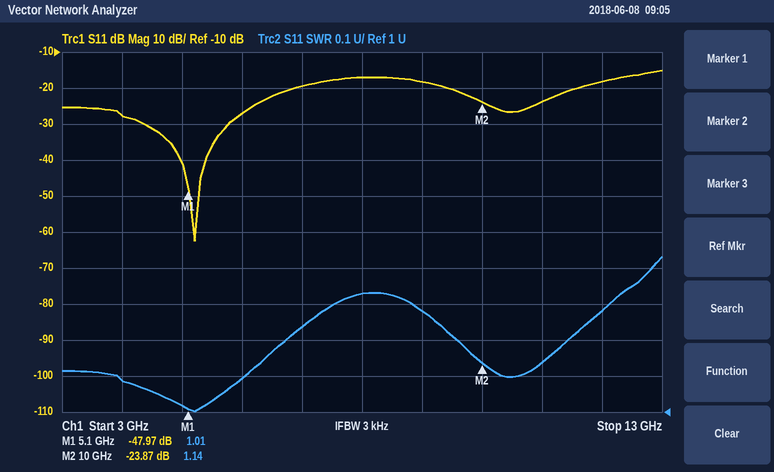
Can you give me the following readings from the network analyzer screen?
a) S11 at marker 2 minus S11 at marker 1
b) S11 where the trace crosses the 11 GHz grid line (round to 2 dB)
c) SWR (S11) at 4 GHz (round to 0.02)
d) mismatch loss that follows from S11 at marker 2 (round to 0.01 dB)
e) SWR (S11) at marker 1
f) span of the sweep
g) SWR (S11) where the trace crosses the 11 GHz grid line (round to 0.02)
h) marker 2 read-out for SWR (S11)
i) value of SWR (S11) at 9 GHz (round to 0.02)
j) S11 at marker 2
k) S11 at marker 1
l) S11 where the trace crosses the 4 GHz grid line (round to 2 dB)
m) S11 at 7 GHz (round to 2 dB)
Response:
24.10 dB
-24 dB
1.08
0.02 dB
1.01
10 GHz
1.14
1.14
1.28
-23.87 dB
-47.97 dB
-28 dB
-20 dB
